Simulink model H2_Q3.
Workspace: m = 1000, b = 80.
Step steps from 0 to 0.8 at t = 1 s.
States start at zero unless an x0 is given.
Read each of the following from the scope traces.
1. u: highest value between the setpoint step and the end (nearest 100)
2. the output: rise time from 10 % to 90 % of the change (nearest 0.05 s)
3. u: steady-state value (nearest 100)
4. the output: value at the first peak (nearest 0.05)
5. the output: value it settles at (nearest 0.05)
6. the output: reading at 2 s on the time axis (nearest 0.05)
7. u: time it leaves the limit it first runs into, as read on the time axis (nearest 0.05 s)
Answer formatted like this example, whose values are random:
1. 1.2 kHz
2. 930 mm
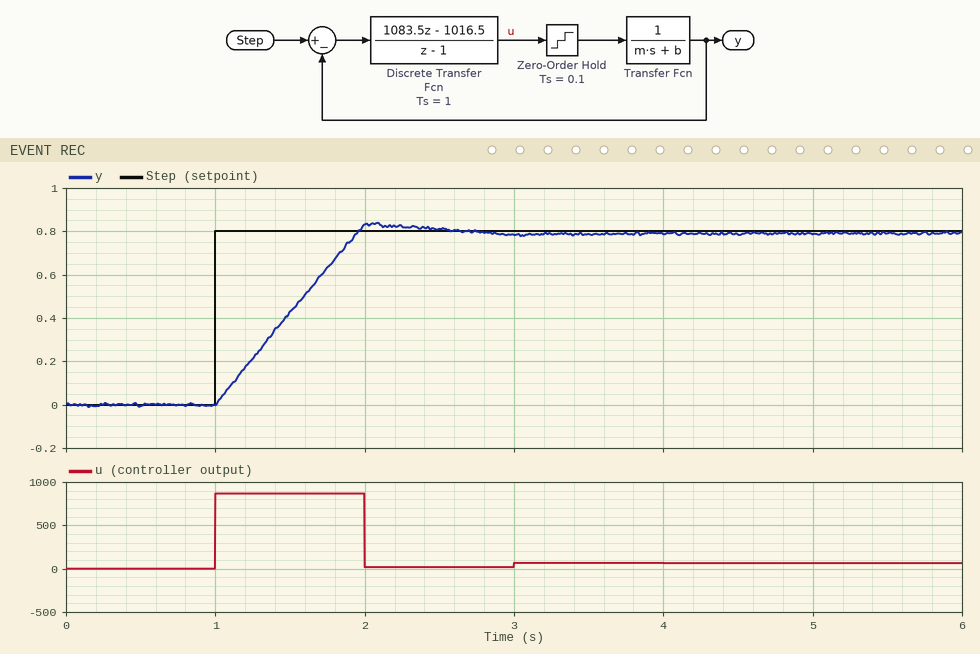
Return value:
1. 900
2. 0.75 s
3. 100
4. 0.85
5. 0.80
6. 0.85
7. 2.00 s
